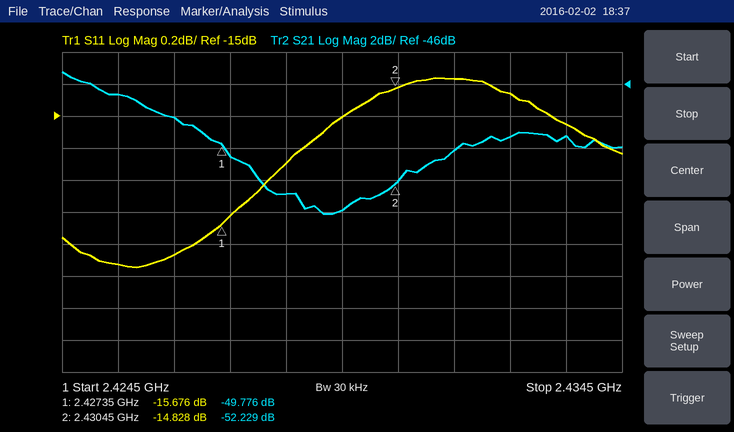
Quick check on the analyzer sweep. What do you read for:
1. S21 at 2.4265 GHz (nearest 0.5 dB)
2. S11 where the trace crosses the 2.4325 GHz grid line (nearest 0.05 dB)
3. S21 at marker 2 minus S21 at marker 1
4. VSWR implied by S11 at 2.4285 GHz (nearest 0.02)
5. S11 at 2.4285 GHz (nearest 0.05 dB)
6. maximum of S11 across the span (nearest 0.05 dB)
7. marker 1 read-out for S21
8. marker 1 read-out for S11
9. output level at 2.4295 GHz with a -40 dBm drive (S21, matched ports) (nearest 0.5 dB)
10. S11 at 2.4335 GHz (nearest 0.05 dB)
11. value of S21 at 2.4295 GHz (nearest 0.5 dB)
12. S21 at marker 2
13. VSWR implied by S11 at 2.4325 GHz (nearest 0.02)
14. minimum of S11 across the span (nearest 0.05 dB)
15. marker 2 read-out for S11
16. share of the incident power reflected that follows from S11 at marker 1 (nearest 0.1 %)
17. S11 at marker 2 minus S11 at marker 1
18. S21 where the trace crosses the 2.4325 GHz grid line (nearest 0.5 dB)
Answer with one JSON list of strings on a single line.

["-48.0 dB", "-14.85 dB", "-2.453 dB", "1.42", "-15.30 dB", "-14.75 dB", "-49.776 dB", "-15.676 dB", "-94.0 dBm", "-15.05 dB", "-54.0 dB", "-52.229 dB", "1.44", "-15.95 dB", "-14.828 dB", "2.7 %", "0.848 dB", "-49.5 dB"]
